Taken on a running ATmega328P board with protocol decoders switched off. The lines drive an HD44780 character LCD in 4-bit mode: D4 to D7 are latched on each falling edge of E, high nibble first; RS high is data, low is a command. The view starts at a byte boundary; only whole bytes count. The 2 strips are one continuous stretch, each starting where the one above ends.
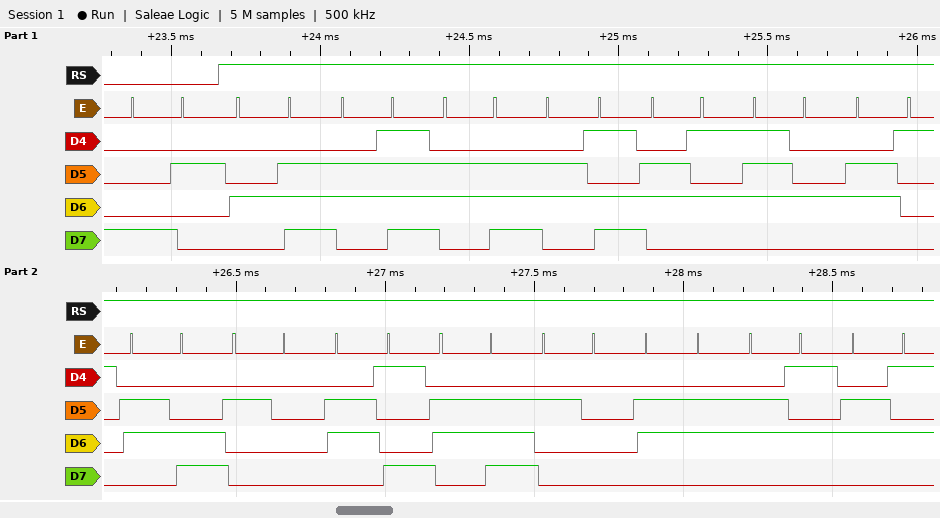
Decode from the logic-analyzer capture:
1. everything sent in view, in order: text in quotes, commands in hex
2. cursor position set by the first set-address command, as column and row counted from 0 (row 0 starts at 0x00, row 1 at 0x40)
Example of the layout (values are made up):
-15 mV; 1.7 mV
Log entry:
0x82 "Nonmetal in fee"; column 2, row 0
